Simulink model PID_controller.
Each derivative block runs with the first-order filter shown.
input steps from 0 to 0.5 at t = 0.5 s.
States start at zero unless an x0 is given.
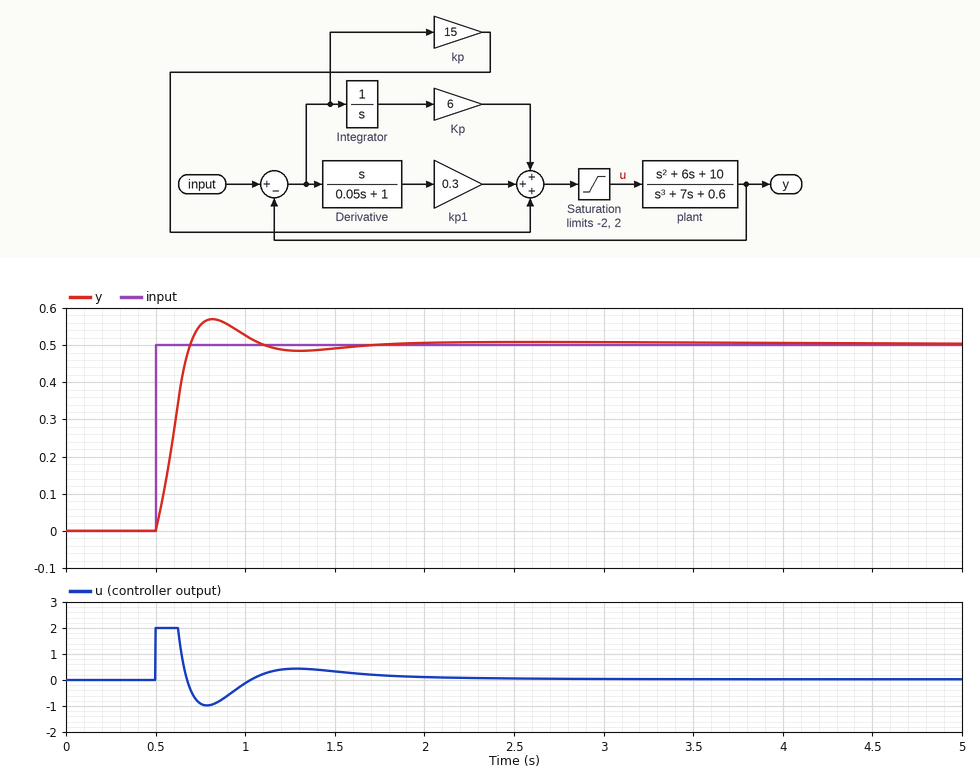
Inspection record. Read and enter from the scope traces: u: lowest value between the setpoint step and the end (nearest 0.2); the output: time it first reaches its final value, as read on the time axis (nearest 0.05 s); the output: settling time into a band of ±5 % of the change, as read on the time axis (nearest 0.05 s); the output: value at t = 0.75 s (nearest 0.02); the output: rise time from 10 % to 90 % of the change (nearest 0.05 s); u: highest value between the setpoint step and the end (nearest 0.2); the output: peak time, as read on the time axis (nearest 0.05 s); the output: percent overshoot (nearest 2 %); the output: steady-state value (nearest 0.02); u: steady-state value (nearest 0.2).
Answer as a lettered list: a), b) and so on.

a) -1.0
b) 0.70 s
c) 1.00 s
d) 0.56
e) 0.15 s
f) 2.0
g) 0.80 s
h) 14 %
i) 0.50
j) 0.0
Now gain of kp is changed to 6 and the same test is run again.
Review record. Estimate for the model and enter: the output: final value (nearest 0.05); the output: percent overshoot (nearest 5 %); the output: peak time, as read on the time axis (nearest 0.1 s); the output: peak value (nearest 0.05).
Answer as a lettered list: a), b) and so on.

a) 0.50
b) 25 %
c) 0.9 s
d) 0.60
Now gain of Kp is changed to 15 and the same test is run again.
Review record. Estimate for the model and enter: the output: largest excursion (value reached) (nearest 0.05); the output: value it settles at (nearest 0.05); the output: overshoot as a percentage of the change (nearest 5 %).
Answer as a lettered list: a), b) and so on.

a) 0.60
b) 0.50
c) 20 %
